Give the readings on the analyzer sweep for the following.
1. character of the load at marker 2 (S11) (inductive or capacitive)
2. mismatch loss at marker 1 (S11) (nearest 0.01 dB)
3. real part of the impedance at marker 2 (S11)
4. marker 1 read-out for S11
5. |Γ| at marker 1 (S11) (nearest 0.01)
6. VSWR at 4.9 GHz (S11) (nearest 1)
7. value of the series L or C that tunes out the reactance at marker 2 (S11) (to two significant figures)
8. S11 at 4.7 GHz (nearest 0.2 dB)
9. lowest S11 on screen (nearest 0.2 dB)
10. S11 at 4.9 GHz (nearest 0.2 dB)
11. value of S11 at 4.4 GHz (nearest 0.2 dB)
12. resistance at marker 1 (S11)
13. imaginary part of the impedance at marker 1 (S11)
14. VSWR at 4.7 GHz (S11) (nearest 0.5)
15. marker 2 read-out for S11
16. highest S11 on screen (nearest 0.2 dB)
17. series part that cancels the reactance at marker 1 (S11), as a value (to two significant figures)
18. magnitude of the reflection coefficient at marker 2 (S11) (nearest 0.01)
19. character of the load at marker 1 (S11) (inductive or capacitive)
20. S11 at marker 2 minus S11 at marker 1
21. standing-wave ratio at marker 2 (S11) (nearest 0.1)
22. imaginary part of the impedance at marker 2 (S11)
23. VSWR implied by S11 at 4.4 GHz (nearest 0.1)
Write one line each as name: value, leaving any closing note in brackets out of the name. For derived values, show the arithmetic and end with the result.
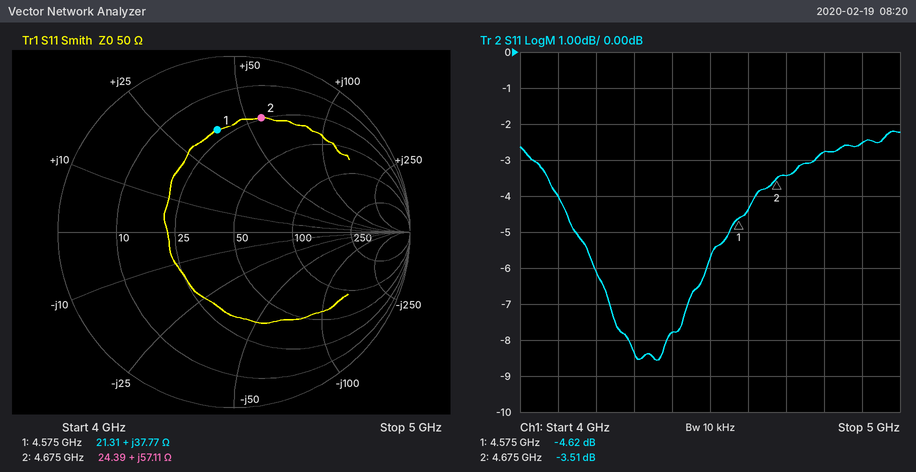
character of the load at marker 2 (S11): inductive
mismatch loss at marker 1 (S11): −10 log10(1 − 10^(-4.62/10)) ≈ 1.84 dB
real part of the impedance at marker 2: 24.39 Ω
marker 1 read-out for S11: -4.62 dB
|Γ| at marker 1 (S11): 0.59
VSWR at 4.9 GHz (S11): |Γ| = 10^(-2.6/20) = 0.7413; VSWR = (1 + 0.7413)/(1 − 0.7413) ≈ 7
value of the series L or C that tunes out the reactance at marker 2 (S11): C = 1/(2π × 4.675 GHz × 57.11 Ω) ≈ 596 fF, so 600 fF to two significant figures
S11 at 4.7 GHz: -3.4 dB
lowest S11 on screen: -8.6 dB
S11 at 4.9 GHz: -2.6 dB
value of S11 at 4.4 GHz: -7.8 dB
resistance at marker 1: 21.31 Ω
imaginary part of the impedance at marker 1: +37.77 Ω
VSWR at 4.7 GHz (S11): |Γ| = 10^(-3.4/20) = 0.6761; VSWR = (1 + 0.6761)/(1 − 0.6761) ≈ 5.17, so 5.0 to the nearest 0.5
marker 2 read-out for S11: -3.51 dB
highest S11 on screen: -2.2 dB
series part that cancels the reactance at marker 1 (S11), as a value: C = 1/(2π × 4.575 GHz × 37.77 Ω) ≈ 921 fF, so 920 fF to two significant figures
magnitude of the reflection coefficient at marker 2 (S11): 10^(-3.51/20) ≈ 0.67
character of the load at marker 1 (S11): inductive
S11 at marker 2 minus S11 at marker 1: -3.51 − (-4.62) = 1.11 dB
standing-wave ratio at marker 2 (S11): 5.0
imaginary part of the impedance at marker 2: +57.11 Ω
VSWR implied by S11 at 4.4 GHz: |Γ| = 10^(-7.8/20) = 0.4074; VSWR = (1 + 0.4074)/(1 − 0.4074) ≈ 2.4
